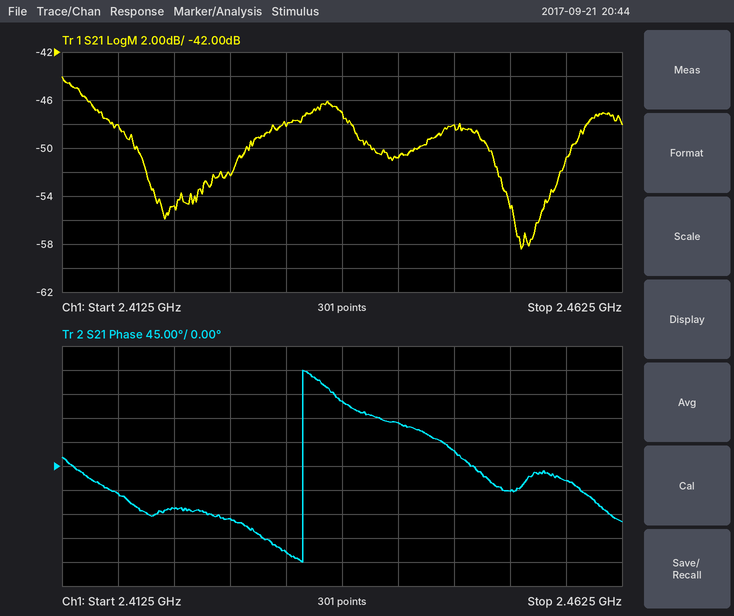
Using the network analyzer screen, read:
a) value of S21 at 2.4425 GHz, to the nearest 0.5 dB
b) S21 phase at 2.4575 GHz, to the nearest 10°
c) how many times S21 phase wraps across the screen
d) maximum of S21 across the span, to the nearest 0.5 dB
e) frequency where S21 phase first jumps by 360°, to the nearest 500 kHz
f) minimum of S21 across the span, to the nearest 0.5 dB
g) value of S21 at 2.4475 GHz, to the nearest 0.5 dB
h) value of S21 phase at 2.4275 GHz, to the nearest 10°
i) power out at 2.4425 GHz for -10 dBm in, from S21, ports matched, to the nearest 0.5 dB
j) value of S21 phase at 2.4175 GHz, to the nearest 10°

-51.0 dB
-30°
1
-44.0 dB
2.4340 GHz
-58.5 dB
-48.0 dB
-100°
-61.0 dBm
-50°
